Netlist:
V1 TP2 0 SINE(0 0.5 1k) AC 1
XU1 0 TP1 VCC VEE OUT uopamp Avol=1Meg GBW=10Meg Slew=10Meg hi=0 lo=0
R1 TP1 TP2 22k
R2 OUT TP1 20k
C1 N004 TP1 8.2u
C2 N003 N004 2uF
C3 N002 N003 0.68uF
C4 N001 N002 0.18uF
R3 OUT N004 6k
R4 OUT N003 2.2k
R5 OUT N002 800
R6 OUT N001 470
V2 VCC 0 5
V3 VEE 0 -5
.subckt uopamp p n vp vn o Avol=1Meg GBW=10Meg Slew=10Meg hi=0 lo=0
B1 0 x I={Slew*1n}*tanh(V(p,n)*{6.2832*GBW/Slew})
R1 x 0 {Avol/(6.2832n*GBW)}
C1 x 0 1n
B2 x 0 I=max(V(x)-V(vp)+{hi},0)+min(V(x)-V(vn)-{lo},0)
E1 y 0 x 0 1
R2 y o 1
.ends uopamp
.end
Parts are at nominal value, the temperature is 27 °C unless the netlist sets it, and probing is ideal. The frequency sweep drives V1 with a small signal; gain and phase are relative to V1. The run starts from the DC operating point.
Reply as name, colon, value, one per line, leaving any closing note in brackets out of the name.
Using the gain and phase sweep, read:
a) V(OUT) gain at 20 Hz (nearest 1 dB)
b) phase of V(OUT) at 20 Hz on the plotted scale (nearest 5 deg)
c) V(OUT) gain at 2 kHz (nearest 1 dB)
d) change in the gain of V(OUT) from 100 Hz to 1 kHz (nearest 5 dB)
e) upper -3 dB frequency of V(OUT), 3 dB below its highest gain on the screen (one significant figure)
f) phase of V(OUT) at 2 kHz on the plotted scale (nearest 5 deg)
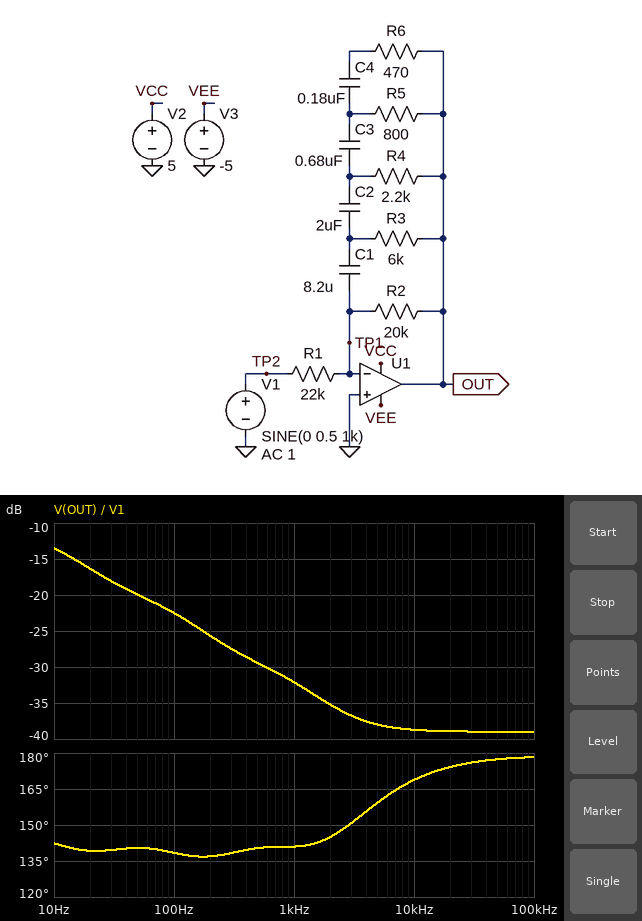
V(OUT) gain at 20 Hz: -16 dB
phase of V(OUT) at 20 Hz on the plotted scale: 140 deg
V(OUT) gain at 2 kHz: -35 dB
change in the gain of V(OUT) from 100 Hz to 1 kHz: -10 dB
upper -3 dB frequency of V(OUT), 3 dB below its highest gain on the screen: 20 Hz
phase of V(OUT) at 2 kHz on the plotted scale: 145 deg
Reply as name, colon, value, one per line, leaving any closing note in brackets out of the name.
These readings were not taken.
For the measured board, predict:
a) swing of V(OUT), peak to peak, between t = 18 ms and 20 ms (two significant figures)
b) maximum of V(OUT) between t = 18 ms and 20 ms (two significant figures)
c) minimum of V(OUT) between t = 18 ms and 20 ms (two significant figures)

swing of V(OUT), peak to peak, between t = 18 ms and 20 ms: 25 mV
maximum of V(OUT) between t = 18 ms and 20 ms: 12 mV
minimum of V(OUT) between t = 18 ms and 20 ms: -13 mV
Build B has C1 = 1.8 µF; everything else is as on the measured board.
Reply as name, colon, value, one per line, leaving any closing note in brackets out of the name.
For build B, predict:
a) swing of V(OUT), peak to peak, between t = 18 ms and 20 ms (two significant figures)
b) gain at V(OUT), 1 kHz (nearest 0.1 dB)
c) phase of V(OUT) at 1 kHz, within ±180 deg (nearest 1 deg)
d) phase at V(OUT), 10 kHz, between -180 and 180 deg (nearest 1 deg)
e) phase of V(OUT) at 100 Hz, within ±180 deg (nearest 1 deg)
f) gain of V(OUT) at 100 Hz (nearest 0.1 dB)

swing of V(OUT), peak to peak, between t = 18 ms and 20 ms: 27 mV
gain at V(OUT), 1 kHz: -31.4 dB
phase of V(OUT) at 1 kHz, within ±180 deg: 136 deg
phase at V(OUT), 10 kHz, between -180 and 180 deg: 167 deg
phase of V(OUT) at 100 Hz, within ±180 deg: 128 deg
gain of V(OUT) at 100 Hz: -20.2 dB
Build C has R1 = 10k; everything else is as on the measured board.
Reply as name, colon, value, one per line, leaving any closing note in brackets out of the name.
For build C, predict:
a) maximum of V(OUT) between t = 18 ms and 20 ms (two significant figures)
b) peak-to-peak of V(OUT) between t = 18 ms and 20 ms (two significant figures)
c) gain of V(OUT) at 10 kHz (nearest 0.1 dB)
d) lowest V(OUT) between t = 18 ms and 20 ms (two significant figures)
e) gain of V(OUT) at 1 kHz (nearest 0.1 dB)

maximum of V(OUT) between t = 18 ms and 20 ms: 26 mV
peak-to-peak of V(OUT) between t = 18 ms and 20 ms: 55 mV
gain of V(OUT) at 10 kHz: -31.9 dB
lowest V(OUT) between t = 18 ms and 20 ms: -28 mV
gain of V(OUT) at 1 kHz: -25.3 dB
